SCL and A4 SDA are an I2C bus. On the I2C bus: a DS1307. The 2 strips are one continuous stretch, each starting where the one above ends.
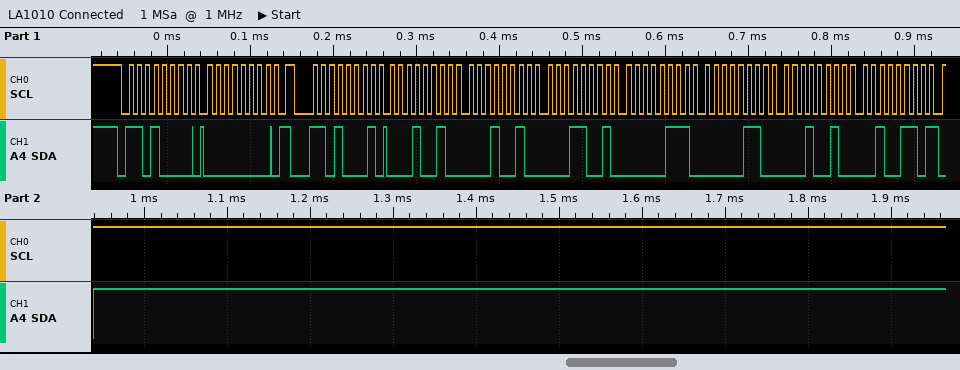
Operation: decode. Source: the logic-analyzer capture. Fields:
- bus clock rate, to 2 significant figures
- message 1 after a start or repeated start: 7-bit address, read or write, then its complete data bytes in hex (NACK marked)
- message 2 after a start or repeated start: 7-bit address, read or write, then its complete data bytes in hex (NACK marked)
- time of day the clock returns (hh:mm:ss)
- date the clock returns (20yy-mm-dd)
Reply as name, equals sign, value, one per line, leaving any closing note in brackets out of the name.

bus clock rate, to 2 significant figures = 100 kHz
message 1 after a start or repeated start: 7-bit address, read or write, then its complete data bytes in hex = 0x68 write: 00
message 2 after a start or repeated start: 7-bit address, read or write, then its complete data bytes in hex = 0x68 read: 12 12 19 07 06 12 26 NACK
time of day the clock returns = 19:12:12
date the clock returns = 2026-12-06
